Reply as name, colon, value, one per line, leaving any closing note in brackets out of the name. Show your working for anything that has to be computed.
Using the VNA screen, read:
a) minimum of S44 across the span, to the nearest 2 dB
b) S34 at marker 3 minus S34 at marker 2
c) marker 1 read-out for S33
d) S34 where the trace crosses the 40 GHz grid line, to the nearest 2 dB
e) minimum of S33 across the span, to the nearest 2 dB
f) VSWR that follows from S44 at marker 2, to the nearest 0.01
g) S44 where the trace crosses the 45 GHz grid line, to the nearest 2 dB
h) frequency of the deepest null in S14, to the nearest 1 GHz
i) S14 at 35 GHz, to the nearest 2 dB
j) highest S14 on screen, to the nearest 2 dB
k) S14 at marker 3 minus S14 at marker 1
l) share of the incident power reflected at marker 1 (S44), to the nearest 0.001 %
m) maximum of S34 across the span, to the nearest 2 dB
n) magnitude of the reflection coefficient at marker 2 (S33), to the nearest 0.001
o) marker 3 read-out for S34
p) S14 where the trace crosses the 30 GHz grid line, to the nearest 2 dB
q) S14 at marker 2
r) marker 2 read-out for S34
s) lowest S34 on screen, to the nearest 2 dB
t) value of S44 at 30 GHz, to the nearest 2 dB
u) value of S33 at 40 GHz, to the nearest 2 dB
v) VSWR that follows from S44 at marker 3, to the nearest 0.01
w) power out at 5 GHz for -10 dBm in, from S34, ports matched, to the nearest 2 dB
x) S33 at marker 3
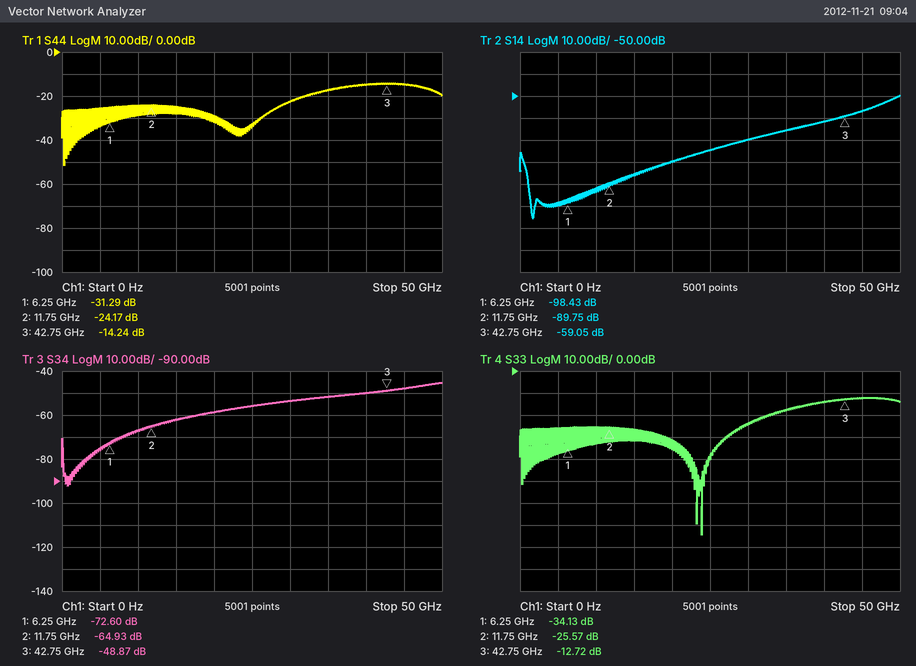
minimum of S44 across the span, to the nearest 2 dB: -52 dB
S34 at marker 3 minus S34 at marker 2: -48.87 − (-64.93) = 16.06 dB
marker 1 read-out for S33: -34.13 dB
S34 where the trace crosses the 40 GHz grid line, to the nearest 2 dB: -50 dB
minimum of S33 across the span, to the nearest 2 dB: -74 dB
VSWR that follows from S44 at marker 2, to the nearest 0.01: (1 + 0.0619)/(1 − 0.0619) ≈ 1.13
S44 where the trace crosses the 45 GHz grid line, to the nearest 2 dB: -14 dB
frequency of the deepest null in S14, to the nearest 1 GHz: 2 GHz
S14 at 35 GHz, to the nearest 2 dB: -66 dB
highest S14 on screen, to the nearest 2 dB: -50 dB
S14 at marker 3 minus S14 at marker 1: -59.05 − (-98.43) = 39.38 dB
share of the incident power reflected at marker 1 (S44), to the nearest 0.001 %: 10^(-31.29/10) ≈ 0.074 %
maximum of S34 across the span, to the nearest 2 dB: -46 dB
magnitude of the reflection coefficient at marker 2 (S33), to the nearest 0.001: 10^(-25.57/20) ≈ 0.053
marker 3 read-out for S34: -48.87 dB
S14 where the trace crosses the 30 GHz grid line, to the nearest 2 dB: -70 dB
S14 at marker 2: -89.75 dB
marker 2 read-out for S34: -64.93 dB
lowest S34 on screen, to the nearest 2 dB: -92 dB
value of S44 at 30 GHz, to the nearest 2 dB: -22 dB
value of S33 at 40 GHz, to the nearest 2 dB: -14 dB
VSWR that follows from S44 at marker 3, to the nearest 0.01: (1 + 0.1941)/(1 − 0.1941) ≈ 1.48
power out at 5 GHz for -10 dBm in, from S34, ports matched, to the nearest 2 dB: -10 dBm + (-76 dB) = -86 dBm
S33 at marker 3: -12.72 dB
